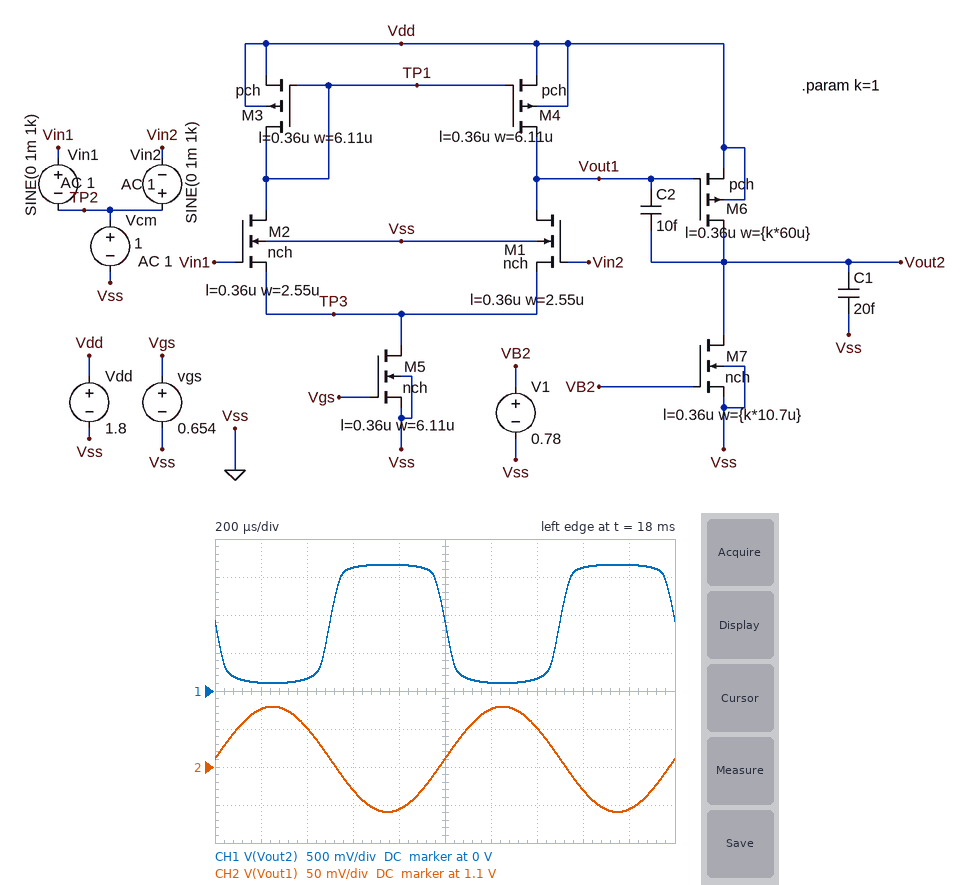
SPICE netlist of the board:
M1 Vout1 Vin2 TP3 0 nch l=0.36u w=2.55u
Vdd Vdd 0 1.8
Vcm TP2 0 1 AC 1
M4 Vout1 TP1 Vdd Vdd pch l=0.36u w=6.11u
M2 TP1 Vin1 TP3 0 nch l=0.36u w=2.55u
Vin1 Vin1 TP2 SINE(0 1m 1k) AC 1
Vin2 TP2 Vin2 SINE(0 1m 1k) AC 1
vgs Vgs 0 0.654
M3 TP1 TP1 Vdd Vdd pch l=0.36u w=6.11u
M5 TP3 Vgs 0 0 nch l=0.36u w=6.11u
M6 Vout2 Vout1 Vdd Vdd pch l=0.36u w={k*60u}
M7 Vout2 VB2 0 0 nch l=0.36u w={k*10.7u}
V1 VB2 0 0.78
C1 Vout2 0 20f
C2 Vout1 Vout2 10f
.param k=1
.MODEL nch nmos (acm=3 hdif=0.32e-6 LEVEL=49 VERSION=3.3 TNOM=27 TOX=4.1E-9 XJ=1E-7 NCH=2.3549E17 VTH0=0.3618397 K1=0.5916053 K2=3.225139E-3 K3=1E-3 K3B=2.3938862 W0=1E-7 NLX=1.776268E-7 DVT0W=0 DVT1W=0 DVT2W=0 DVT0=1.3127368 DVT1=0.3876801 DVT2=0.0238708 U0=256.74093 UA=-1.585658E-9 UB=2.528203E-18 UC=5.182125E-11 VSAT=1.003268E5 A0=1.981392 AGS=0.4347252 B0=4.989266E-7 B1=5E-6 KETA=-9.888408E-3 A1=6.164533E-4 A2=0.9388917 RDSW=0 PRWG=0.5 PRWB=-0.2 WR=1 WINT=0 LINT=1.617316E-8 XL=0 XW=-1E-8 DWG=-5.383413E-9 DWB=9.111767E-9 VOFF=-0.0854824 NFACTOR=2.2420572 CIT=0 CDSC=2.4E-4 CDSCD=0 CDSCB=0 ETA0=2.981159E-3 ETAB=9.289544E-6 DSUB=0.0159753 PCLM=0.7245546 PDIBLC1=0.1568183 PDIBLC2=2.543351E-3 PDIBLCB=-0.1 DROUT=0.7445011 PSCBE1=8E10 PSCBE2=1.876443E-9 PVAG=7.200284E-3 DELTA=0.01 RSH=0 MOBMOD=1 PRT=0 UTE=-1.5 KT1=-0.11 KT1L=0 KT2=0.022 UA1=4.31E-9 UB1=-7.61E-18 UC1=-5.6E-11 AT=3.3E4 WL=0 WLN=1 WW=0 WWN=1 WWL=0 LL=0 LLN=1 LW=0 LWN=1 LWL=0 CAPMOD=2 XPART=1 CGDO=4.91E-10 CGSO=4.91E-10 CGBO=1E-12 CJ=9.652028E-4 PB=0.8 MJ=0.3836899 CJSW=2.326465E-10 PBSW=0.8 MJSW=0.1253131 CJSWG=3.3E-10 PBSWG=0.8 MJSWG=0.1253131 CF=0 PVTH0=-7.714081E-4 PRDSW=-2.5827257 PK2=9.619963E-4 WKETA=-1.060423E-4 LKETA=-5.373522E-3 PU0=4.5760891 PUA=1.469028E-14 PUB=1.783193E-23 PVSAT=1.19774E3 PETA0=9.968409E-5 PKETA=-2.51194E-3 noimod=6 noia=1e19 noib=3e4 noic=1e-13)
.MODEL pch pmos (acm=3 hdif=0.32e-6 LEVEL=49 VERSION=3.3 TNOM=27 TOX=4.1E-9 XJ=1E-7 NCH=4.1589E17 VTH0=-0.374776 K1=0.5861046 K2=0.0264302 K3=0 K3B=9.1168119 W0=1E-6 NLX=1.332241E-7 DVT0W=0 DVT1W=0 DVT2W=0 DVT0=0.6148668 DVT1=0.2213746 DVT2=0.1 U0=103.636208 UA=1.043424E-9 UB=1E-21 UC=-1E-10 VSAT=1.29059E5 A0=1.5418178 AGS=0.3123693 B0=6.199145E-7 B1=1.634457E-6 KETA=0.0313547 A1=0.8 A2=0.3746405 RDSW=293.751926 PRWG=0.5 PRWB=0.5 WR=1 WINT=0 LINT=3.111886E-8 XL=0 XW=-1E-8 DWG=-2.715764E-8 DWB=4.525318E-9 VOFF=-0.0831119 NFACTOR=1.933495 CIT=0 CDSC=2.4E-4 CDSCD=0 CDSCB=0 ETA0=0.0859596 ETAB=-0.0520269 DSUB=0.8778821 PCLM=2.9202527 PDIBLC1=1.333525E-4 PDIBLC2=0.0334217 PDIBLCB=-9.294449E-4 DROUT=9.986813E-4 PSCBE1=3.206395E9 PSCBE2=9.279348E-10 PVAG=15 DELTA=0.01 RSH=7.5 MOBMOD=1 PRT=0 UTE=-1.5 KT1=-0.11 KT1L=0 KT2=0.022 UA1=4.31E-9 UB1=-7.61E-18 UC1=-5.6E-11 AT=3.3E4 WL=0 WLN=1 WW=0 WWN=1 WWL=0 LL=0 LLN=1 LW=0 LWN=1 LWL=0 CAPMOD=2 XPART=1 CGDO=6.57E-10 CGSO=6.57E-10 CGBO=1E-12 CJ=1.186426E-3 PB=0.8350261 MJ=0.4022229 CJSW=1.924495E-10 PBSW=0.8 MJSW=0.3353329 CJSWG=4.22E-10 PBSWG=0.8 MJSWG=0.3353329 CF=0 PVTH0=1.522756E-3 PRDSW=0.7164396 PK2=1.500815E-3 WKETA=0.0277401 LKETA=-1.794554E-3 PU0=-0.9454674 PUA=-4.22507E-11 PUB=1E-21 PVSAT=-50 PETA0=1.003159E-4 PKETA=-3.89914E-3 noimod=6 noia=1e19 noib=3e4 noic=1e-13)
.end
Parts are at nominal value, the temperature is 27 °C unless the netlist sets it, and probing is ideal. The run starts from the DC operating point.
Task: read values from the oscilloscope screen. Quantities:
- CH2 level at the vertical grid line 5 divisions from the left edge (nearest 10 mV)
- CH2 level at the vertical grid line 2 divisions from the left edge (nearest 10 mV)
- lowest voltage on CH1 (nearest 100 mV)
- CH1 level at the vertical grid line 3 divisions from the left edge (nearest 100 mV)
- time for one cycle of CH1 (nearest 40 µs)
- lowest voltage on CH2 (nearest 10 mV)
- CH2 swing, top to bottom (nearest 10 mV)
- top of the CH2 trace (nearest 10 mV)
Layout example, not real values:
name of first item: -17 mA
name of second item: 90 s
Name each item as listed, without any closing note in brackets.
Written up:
CH2 level at the vertical grid line 5 divisions from the left edge: 1.11 V
CH2 level at the vertical grid line 2 divisions from the left edge: 1.15 V
lowest voltage on CH1: 100 mV
CH1 level at the vertical grid line 3 divisions from the left edge: 1.6 V
time for one cycle of CH1: 1.00 ms
lowest voltage on CH2: 1.04 V
CH2 swing, top to bottom: 140 mV
top of the CH2 trace: 1.18 V
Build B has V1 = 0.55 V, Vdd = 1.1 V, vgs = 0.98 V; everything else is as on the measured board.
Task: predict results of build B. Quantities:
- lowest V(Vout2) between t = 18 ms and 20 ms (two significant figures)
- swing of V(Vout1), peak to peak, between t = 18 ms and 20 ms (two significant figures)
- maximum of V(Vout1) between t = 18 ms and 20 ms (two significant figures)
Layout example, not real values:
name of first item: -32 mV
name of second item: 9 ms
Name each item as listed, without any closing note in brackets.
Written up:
lowest V(Vout2) between t = 18 ms and 20 ms: 1.1 V
swing of V(Vout1), peak to peak, between t = 18 ms and 20 ms: 2.2 mV
maximum of V(Vout1) between t = 18 ms and 20 ms: 240 mV
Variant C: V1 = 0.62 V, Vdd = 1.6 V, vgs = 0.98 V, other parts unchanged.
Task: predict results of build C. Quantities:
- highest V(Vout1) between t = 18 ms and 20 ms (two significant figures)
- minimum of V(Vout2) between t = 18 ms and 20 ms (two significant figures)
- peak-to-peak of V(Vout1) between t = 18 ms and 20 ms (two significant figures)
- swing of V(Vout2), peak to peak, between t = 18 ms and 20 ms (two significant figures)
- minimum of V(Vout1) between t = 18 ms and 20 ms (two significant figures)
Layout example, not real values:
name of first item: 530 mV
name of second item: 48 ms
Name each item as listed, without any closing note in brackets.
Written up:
highest V(Vout1) between t = 18 ms and 20 ms: 720 mV
minimum of V(Vout2) between t = 18 ms and 20 ms: 1.6 V
peak-to-peak of V(Vout1) between t = 18 ms and 20 ms: 84 mV
swing of V(Vout2), peak to peak, between t = 18 ms and 20 ms: 3.2 mV
minimum of V(Vout1) between t = 18 ms and 20 ms: 640 mV
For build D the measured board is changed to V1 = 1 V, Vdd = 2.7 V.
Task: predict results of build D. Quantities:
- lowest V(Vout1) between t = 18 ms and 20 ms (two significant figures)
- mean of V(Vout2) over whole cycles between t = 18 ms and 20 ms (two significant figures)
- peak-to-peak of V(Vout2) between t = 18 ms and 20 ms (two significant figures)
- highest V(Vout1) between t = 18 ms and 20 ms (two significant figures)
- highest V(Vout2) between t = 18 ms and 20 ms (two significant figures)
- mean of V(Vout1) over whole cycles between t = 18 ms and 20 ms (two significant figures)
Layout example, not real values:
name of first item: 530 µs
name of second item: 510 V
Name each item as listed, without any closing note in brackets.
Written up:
lowest V(Vout1) between t = 18 ms and 20 ms: 1.9 V
mean of V(Vout2) over whole cycles between t = 18 ms and 20 ms: 120 mV
peak-to-peak of V(Vout2) between t = 18 ms and 20 ms: 160 mV
highest V(Vout1) between t = 18 ms and 20 ms: 2.1 V
highest V(Vout2) between t = 18 ms and 20 ms: 210 mV
mean of V(Vout1) over whole cycles between t = 18 ms and 20 ms: 2.0 V
